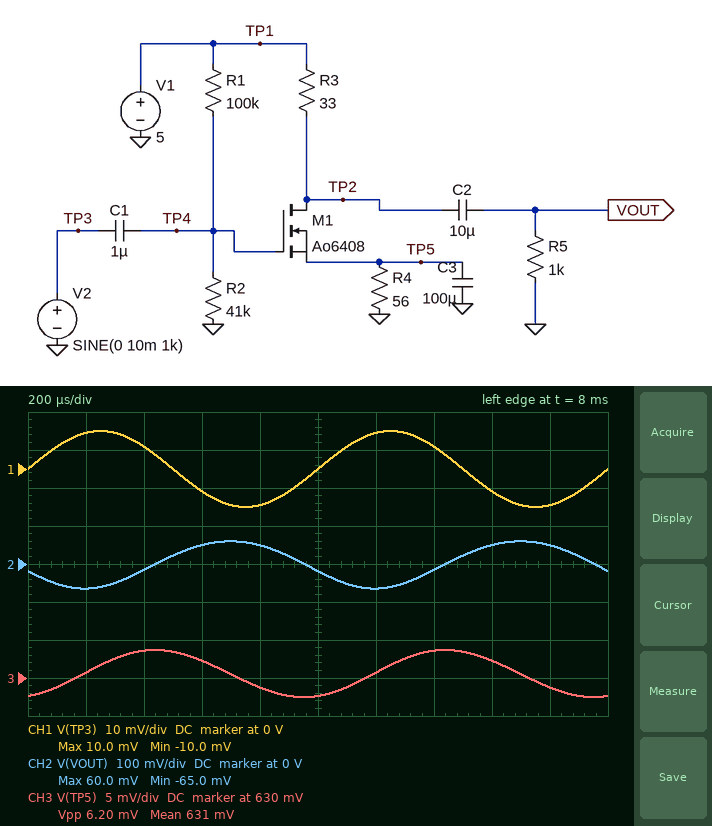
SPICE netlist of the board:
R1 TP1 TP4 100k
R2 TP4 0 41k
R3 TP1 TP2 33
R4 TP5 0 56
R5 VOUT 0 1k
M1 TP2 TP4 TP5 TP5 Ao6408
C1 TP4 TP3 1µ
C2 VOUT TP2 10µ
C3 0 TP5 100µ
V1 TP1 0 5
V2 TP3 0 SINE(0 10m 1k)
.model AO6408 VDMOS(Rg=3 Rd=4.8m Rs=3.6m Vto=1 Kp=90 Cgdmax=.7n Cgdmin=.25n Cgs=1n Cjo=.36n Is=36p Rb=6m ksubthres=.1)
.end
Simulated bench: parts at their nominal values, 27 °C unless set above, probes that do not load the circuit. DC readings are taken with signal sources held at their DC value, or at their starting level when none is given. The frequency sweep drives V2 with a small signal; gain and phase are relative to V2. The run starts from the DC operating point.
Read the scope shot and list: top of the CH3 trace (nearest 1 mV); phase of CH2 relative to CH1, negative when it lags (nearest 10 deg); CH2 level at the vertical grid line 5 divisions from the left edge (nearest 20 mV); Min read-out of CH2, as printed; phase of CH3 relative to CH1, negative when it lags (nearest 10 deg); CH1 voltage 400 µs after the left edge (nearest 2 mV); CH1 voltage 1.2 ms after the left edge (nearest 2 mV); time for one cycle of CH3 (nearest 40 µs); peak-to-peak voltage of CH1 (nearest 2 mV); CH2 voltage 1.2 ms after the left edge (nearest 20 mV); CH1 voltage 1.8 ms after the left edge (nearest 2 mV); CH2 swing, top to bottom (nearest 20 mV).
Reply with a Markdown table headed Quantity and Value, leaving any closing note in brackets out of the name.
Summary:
| Quantity | Value |
|---|---|
| top of the CH3 trace | 634 mV |
| phase of CH2 relative to CH1, negative when it lags | -160 deg |
| CH2 level at the vertical grid line 5 divisions from the left edge | -20 mV |
| Min read-out of CH2, as printed | -65.0 mV |
| phase of CH3 relative to CH1, negative when it lags | -70 deg |
| CH1 voltage 400 µs after the left edge | 6 mV |
| CH1 voltage 1.2 ms after the left edge | 10 mV |
| time for one cycle of CH3 | 1.00 ms |
| peak-to-peak voltage of CH1 | 20 mV |
| CH2 voltage 1.2 ms after the left edge | -60 mV |
| CH1 voltage 1.8 ms after the left edge | -10 mV |
| CH2 swing, top to bottom | 120 mV |
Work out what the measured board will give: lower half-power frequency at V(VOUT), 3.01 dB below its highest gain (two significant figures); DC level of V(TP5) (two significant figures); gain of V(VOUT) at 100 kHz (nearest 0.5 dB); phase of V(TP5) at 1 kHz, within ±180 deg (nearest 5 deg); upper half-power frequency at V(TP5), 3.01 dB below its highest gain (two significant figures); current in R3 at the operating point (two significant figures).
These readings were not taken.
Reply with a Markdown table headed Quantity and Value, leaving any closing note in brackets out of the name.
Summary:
| Quantity | Value |
|---|---|
| lower half-power frequency at V(VOUT), 3.01 dB below its highest gain | 360 Hz |
| DC level of V(TP5) | 630 mV |
| gain of V(VOUT) at 100 kHz | 16.5 dB |
| phase of V(TP5) at 1 kHz, within ±180 deg | -70 deg |
| upper half-power frequency at V(TP5), 3.01 dB below its highest gain | 370 Hz |
| current in R3 at the operating point | 11 mA |
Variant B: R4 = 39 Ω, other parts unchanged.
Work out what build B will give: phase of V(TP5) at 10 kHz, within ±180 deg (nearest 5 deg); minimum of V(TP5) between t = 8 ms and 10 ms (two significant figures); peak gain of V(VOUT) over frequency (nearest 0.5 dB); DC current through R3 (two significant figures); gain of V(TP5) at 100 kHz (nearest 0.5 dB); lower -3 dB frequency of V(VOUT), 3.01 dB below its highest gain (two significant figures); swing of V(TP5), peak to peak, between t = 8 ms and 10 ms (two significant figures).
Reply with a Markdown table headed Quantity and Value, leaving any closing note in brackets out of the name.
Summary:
| Quantity | Value |
|---|---|
| phase of V(TP5) at 10 kHz, within ±180 deg | -85 deg |
| minimum of V(TP5) between t = 8 ms and 10 ms | 610 mV |
| peak gain of V(VOUT) over frequency | 19.0 dB |
| DC current through R3 | 16 mA |
| gain of V(TP5) at 100 kHz | -47.0 dB |
| lower -3 dB frequency of V(VOUT), 3.01 dB below its highest gain | 490 Hz |
| swing of V(TP5), peak to peak, between t = 8 ms and 10 ms | 8.1 mV |
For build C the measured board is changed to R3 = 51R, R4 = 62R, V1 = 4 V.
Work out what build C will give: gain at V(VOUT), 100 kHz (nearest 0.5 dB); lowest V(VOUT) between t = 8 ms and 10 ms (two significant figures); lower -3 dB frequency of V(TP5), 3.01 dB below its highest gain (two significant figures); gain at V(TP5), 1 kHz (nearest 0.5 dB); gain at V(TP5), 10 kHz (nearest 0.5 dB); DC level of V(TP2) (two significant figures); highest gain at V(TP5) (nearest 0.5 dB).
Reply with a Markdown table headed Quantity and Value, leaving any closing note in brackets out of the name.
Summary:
| Quantity | Value |
|---|---|
| gain at V(VOUT), 100 kHz | 15.0 dB |
| lowest V(VOUT) between t = 8 ms and 10 ms | -56 mV |
| lower -3 dB frequency of V(TP5), 3.01 dB below its highest gain | 5.2 Hz |
| gain at V(TP5), 1 kHz | -15.0 dB |
| gain at V(TP5), 10 kHz | -35.0 dB |
| DC level of V(TP2) | 3.7 V |
| highest gain at V(TP5) | -1.5 dB |
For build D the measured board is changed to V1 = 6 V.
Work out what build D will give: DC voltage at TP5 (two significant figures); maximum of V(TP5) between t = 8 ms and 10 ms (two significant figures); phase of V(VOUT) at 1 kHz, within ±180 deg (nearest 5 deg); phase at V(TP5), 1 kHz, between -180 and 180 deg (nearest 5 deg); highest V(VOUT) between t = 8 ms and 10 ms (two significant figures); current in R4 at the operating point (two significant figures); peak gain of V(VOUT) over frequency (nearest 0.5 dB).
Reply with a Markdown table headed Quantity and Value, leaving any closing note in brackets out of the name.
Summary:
| Quantity | Value |
|---|---|
| DC voltage at TP5 | 900 mV |
| maximum of V(TP5) between t = 8 ms and 10 ms | 910 mV |
| phase of V(VOUT) at 1 kHz, within ±180 deg | -155 deg |
| phase at V(TP5), 1 kHz, between -180 and 180 deg | -65 deg |
| highest V(VOUT) between t = 8 ms and 10 ms | 80 mV |
| current in R4 at the operating point | 16 mA |
| peak gain of V(VOUT) over frequency | 19.5 dB |
